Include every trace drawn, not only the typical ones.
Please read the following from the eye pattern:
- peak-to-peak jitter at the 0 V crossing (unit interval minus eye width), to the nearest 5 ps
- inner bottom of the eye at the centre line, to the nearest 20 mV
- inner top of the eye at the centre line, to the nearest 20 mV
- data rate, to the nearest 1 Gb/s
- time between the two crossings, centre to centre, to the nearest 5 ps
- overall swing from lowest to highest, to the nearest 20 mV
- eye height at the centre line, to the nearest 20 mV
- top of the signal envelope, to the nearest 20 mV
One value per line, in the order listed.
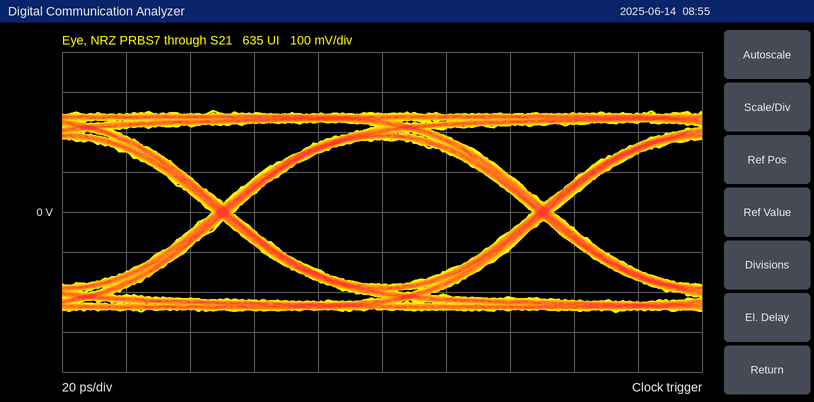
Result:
5 ps
-180 mV
180 mV
10 Gb/s
100 ps
500 mV
360 mV
260 mV
